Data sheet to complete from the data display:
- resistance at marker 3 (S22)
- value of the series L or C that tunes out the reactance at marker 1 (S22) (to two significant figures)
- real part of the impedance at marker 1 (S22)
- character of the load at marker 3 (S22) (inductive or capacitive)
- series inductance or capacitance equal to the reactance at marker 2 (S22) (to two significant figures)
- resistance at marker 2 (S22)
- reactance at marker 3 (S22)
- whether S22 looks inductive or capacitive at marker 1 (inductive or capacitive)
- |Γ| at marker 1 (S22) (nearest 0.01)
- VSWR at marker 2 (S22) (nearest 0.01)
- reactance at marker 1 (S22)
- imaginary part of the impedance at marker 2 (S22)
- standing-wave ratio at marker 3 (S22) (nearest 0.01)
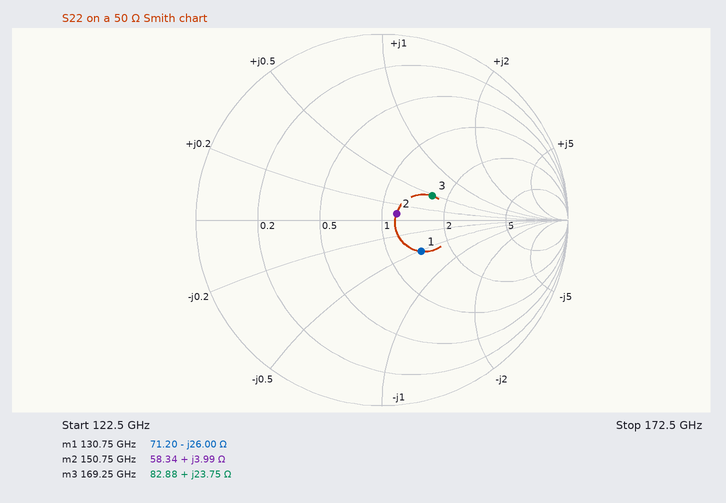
82.88 Ω
32 pH
71.20 Ω
inductive
4.2 pH
58.34 Ω
+23.75 Ω
capacitive
0.27
1.19
-26.00 Ω
+3.99 Ω
1.86
